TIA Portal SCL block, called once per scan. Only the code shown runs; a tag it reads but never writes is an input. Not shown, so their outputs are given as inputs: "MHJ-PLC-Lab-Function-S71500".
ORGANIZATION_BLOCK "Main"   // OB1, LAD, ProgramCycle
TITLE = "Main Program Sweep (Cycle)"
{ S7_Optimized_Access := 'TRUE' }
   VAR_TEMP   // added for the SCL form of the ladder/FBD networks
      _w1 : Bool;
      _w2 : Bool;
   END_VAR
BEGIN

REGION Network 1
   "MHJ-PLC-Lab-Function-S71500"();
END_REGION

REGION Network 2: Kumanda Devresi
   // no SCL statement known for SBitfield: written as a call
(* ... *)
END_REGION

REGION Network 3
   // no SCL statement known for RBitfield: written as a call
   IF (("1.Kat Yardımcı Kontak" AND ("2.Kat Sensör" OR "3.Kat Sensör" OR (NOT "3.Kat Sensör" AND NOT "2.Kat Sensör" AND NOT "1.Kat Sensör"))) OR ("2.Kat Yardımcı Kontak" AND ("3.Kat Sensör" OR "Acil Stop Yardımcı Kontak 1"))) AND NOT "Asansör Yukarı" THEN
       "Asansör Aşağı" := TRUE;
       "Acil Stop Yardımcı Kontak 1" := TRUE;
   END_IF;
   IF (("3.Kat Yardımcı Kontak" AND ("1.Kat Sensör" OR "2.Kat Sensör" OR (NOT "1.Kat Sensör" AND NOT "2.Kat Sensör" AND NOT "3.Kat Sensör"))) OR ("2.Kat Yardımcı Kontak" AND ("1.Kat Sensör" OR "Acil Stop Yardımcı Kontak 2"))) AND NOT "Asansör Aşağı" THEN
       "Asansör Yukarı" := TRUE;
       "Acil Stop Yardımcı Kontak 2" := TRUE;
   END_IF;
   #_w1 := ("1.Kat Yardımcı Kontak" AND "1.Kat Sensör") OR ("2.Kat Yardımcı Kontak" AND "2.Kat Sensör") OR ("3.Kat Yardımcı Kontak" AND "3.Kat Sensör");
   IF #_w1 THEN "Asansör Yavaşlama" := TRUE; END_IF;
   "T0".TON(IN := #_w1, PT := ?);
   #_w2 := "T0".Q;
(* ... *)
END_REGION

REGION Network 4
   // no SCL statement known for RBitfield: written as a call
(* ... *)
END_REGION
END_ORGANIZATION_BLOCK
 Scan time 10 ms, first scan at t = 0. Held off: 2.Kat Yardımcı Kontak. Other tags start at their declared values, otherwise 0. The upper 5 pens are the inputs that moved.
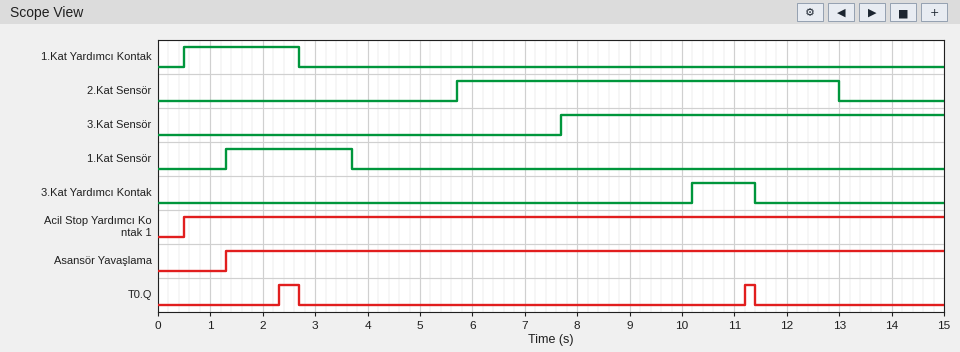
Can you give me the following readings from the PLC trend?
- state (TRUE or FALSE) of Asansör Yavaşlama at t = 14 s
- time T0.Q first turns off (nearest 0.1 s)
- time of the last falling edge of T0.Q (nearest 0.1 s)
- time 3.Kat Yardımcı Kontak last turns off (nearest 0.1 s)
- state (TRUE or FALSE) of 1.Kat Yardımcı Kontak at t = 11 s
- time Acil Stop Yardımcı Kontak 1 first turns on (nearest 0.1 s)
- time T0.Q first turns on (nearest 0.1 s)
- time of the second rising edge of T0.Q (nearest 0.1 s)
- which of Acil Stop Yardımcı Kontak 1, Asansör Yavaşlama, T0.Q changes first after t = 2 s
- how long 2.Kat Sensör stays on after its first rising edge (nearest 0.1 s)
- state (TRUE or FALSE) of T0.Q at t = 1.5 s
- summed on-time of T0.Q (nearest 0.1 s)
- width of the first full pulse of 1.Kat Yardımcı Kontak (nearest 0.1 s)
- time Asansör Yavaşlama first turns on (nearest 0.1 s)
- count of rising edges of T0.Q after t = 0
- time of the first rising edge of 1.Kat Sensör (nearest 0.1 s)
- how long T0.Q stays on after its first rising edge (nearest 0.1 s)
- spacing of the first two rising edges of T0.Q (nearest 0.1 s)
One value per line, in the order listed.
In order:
TRUE
2.7 s
11.4 s
11.4 s
FALSE
0.5 s
2.3 s
11.2 s
T0.Q
7.3 s
FALSE
0.6 s
2.2 s
1.3 s
2
1.3 s
0.4 s
8.9 s
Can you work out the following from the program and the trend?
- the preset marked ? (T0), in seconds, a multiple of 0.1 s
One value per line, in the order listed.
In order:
1.0 s
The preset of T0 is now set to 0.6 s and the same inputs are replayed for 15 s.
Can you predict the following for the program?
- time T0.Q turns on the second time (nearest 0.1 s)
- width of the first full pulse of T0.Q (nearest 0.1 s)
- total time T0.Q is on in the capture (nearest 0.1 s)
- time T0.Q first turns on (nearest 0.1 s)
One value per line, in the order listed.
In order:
10.8 s
0.8 s
1.4 s
1.9 s
